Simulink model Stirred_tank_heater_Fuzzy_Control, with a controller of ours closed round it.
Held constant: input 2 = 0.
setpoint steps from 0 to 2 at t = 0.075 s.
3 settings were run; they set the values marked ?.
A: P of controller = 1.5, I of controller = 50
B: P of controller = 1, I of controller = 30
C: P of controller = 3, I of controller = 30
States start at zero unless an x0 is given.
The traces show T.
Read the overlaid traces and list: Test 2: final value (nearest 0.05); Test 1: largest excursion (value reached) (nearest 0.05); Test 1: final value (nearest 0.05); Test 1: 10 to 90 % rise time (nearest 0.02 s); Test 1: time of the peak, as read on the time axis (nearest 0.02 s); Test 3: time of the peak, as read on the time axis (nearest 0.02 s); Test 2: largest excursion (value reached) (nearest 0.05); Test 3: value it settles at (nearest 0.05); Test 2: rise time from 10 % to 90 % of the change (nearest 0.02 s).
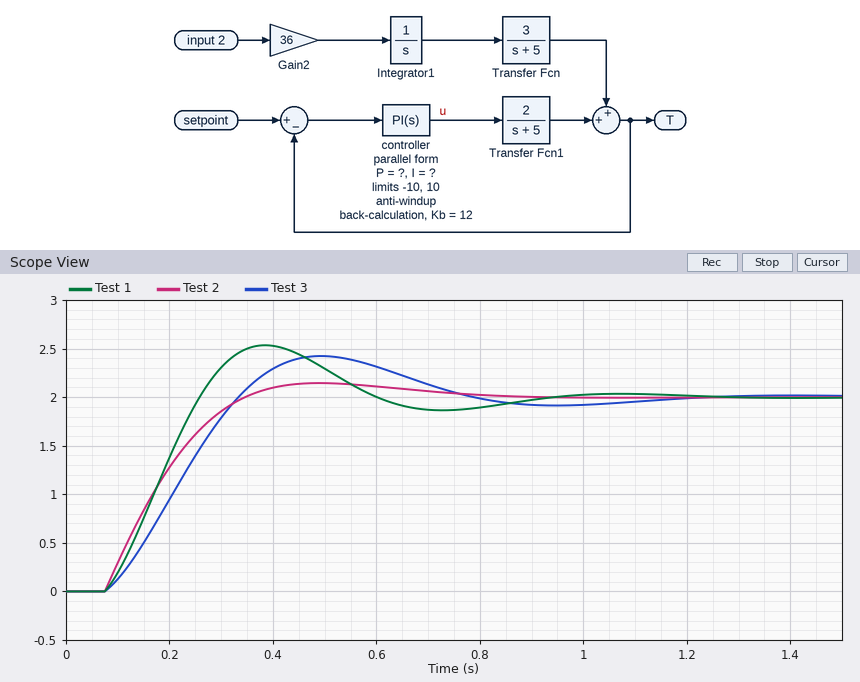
2.00
2.55
2.00
0.14 s
0.38 s
0.50 s
2.15
2.00
0.20 s
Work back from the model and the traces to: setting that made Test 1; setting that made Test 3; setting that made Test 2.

A
B
C
